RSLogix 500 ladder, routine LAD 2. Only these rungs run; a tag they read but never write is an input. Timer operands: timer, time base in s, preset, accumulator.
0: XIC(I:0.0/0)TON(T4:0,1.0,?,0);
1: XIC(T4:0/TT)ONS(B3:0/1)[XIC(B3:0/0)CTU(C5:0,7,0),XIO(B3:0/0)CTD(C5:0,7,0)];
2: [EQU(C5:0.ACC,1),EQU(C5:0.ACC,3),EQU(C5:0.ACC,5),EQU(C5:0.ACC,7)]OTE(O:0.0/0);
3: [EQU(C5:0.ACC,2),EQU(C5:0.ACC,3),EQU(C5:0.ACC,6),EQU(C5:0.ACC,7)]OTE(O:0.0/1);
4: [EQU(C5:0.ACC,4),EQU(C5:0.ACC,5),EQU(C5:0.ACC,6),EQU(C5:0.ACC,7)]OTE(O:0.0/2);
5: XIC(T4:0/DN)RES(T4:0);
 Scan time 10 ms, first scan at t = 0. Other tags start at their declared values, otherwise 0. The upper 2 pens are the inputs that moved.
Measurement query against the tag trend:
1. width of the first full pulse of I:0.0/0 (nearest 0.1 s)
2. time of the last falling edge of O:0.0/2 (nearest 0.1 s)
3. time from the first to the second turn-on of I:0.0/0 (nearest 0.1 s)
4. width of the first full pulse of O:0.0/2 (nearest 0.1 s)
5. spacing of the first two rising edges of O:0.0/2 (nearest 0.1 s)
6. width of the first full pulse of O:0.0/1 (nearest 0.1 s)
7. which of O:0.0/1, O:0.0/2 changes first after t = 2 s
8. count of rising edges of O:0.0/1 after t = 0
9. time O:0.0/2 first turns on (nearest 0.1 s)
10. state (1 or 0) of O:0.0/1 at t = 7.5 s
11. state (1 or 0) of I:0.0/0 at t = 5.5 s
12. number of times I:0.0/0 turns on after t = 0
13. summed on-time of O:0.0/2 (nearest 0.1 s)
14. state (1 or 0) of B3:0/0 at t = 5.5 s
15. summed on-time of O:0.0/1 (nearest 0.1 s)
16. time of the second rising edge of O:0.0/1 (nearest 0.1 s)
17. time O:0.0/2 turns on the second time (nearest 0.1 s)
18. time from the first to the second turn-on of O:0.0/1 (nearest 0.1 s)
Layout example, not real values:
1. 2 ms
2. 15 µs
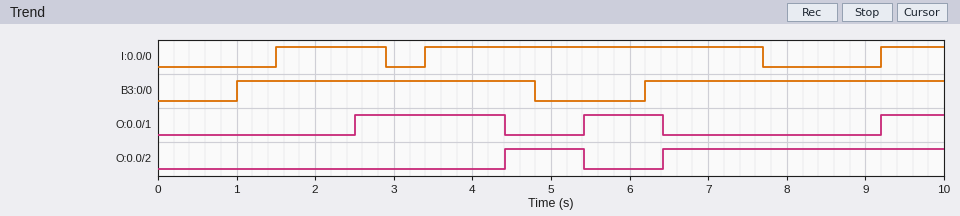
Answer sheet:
1. 1.4 s
2. 5.4 s
3. 1.9 s
4. 1.0 s
5. 2.0 s
6. 1.9 s
7. O:0.0/1
8. 3
9. 4.4 s
10. 0
11. 1
12. 3
13. 4.6 s
14. 0
15. 3.7 s
16. 5.4 s
17. 6.4 s
18. 2.9 s
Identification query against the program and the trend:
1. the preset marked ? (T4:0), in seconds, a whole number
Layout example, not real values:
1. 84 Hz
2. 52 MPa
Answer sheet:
1. 1 s
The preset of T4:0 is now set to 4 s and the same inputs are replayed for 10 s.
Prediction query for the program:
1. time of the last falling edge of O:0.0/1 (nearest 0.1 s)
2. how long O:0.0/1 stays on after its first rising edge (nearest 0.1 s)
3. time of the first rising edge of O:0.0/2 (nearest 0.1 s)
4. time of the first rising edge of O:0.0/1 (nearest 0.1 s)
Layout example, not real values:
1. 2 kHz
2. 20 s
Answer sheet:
1. 9.2 s
2. 5.8 s
3. 9.2 s
4. 3.4 s
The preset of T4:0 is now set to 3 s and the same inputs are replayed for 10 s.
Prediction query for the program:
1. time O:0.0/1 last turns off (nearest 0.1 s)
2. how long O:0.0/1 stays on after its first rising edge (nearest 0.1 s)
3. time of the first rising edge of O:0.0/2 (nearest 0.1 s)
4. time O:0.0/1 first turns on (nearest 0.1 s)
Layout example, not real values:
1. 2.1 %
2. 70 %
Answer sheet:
1. 9.2 s
2. 5.8 s
3. 9.2 s
4. 3.4 s
